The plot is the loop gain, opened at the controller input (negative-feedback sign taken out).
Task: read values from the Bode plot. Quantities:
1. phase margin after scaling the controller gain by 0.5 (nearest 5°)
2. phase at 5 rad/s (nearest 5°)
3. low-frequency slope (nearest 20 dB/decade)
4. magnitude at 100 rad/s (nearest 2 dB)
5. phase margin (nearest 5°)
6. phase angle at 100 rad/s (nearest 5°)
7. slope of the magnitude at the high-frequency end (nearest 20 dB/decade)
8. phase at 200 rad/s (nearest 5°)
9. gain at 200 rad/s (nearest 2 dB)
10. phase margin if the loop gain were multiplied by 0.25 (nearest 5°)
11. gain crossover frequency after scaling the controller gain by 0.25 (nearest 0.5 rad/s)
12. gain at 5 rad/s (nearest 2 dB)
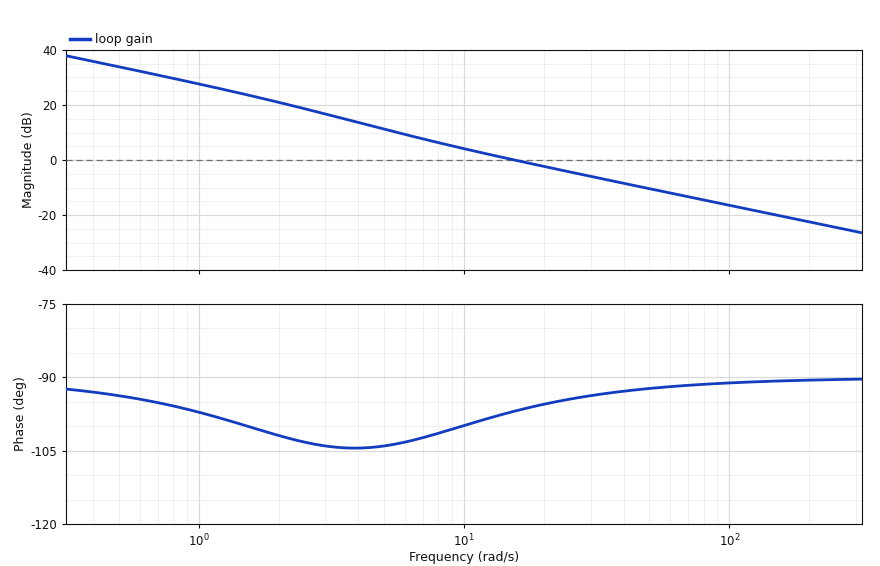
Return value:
80°
-105°
-20 dB/decade
-16 dB
85°
-90°
-20 dB/decade
-90°
-22 dB
75°
4.5 rad/s
12 dB
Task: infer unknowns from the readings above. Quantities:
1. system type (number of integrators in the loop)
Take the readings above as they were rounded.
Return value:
1
